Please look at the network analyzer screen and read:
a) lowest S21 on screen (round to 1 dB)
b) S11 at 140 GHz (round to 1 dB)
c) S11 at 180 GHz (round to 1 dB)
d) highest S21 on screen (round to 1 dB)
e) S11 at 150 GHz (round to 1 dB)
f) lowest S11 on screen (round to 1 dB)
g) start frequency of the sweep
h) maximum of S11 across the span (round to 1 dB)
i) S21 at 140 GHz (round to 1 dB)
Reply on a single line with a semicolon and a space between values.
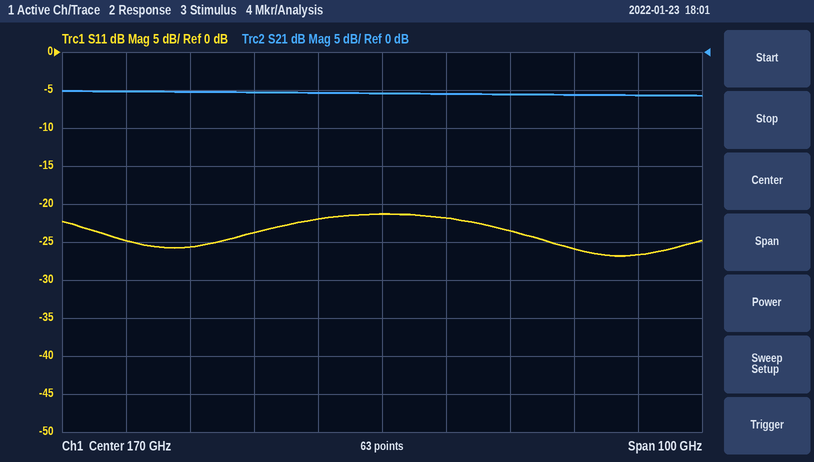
-6 dB; -26 dB; -22 dB; -5 dB; -24 dB; -27 dB; 120 GHz; -21 dB; -5 dB
